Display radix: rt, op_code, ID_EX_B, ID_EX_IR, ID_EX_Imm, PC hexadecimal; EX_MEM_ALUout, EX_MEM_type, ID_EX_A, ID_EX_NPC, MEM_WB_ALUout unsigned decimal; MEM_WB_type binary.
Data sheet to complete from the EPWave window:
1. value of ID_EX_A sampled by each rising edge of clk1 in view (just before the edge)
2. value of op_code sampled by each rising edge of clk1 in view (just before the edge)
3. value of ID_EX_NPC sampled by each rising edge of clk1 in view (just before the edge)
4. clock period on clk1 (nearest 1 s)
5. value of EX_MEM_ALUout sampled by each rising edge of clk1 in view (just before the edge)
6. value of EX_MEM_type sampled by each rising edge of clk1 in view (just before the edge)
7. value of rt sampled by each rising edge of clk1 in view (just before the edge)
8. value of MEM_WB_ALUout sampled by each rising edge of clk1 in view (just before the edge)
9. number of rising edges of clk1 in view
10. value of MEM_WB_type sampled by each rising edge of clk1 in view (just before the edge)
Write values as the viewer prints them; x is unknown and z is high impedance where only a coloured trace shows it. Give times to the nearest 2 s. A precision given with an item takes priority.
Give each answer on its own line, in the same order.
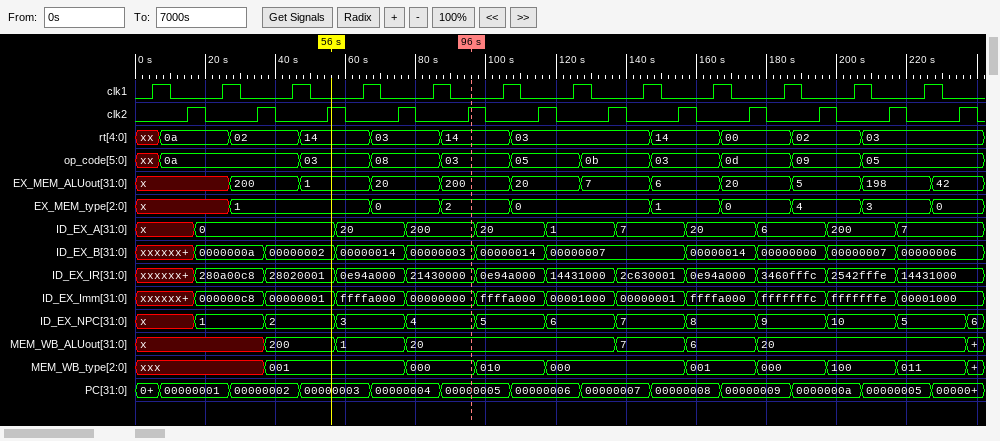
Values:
x, 0, 0, 20, 200, 20, 1, 7, 20, 6, 200, 7
xx, 0a, 0a, 03, 08, 03, 05, 0b, 03, 0d, 09, 05
x, 1, 2, 3, 4, 5, 6, 7, 8, 9, 10, 5
20 s
x, x, 200, 1, 20, 200, 20, 7, 6, 20, 5, 198
x, x, 1, 1, 0, 2, 0, 0, 1, 0, 4, 3
xx, 0a, 02, 14, 03, 14, 03, 03, 14, 00, 02, 03
x, x, 200, 1, 20, 20, 20, 7, 6, 20, 20, 20
12
xxx, xxx, 001, 001, 000, 010, 000, 000, 001, 000, 100, 011
